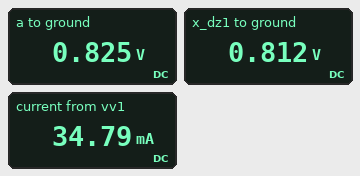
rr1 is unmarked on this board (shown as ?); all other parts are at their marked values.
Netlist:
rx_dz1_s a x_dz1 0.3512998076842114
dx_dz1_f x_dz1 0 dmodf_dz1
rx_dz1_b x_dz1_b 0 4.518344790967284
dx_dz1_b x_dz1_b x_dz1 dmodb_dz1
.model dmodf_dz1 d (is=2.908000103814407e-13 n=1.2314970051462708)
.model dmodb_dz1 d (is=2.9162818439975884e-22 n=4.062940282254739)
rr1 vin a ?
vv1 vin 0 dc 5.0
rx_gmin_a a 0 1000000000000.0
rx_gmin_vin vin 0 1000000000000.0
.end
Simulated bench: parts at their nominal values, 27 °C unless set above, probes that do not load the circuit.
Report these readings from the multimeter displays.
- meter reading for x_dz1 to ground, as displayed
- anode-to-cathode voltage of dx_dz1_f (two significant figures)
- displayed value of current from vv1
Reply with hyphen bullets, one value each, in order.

- 0.812 V
- 810 mV
- 34.79 mA
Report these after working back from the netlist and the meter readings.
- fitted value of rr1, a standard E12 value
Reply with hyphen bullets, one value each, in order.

- 120 Ω
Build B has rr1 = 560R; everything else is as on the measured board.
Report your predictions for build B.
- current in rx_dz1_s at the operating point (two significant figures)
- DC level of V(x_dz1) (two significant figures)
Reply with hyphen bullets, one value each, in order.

- 7.6 mA
- 760 mV
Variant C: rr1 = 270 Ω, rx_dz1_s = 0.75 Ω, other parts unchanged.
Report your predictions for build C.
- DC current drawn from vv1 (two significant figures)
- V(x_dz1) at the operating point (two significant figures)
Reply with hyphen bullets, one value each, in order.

- 16 mA
- 790 mV
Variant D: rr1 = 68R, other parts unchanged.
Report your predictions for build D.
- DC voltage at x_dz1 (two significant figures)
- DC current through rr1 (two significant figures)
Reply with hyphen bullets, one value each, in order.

- 830 mV
- 61 mA
